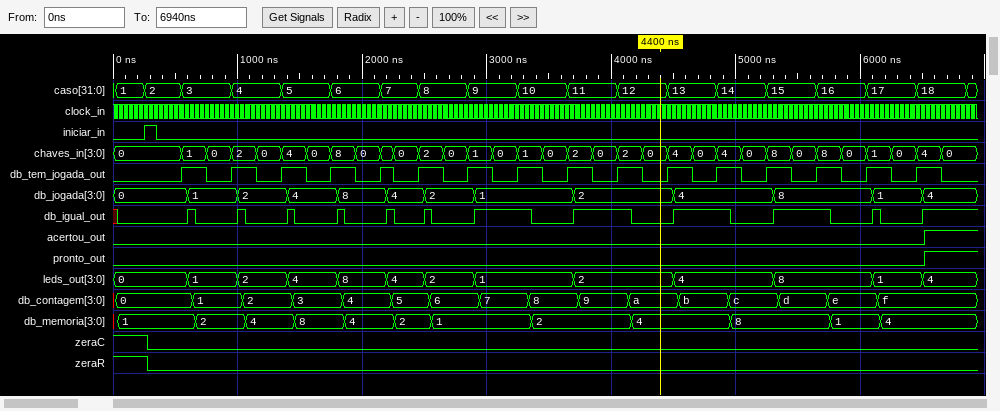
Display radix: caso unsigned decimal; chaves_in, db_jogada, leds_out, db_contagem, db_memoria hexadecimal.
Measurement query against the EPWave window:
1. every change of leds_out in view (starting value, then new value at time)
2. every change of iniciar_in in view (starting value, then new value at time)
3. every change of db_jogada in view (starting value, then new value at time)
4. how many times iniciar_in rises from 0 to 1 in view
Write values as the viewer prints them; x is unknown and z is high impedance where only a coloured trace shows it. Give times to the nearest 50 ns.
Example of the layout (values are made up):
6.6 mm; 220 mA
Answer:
0, 1 at 600 ns, 2 at 1000 ns, 4 at 1400 ns, 8 at 1800 ns, 4 at 2200 ns, 2 at 2500 ns, 1 at 2900 ns, 2 at 3700 ns, 4 at 4500 ns, 8 at 5300 ns, 1 at 6100 ns, 4 at 6500 ns; 0, 1 at 250 ns, 0 at 350 ns; 0, 1 at 600 ns, 2 at 1000 ns, 4 at 1400 ns, 8 at 1800 ns, 4 at 2200 ns, 2 at 2500 ns, 1 at 2900 ns, 2 at 3700 ns, 4 at 4500 ns, 8 at 5300 ns, 1 at 6100 ns, 4 at 6500 ns; 1
